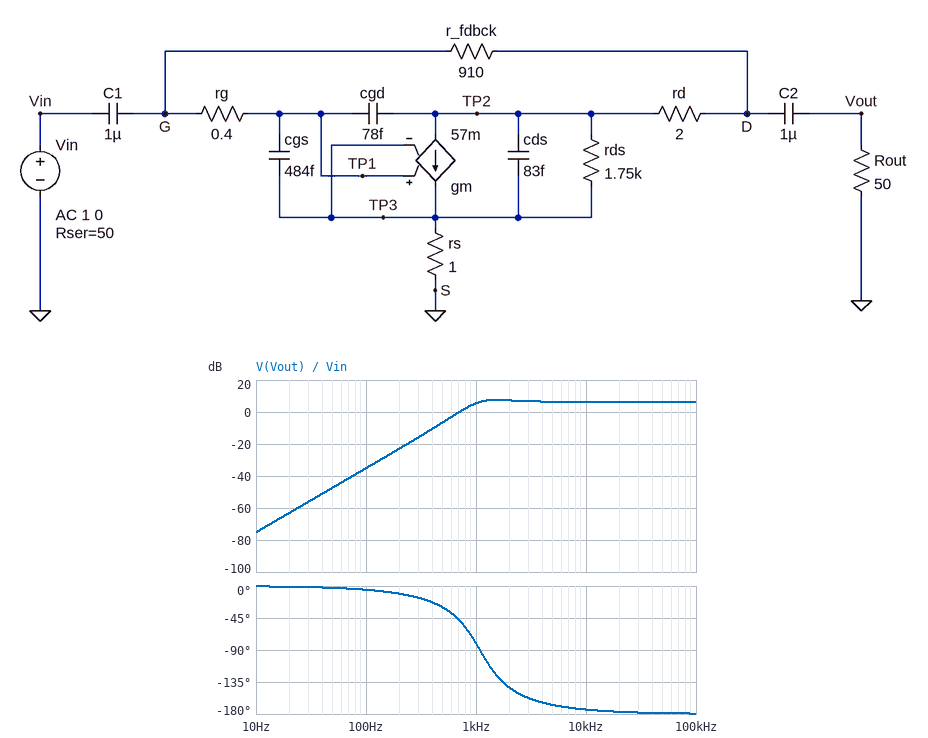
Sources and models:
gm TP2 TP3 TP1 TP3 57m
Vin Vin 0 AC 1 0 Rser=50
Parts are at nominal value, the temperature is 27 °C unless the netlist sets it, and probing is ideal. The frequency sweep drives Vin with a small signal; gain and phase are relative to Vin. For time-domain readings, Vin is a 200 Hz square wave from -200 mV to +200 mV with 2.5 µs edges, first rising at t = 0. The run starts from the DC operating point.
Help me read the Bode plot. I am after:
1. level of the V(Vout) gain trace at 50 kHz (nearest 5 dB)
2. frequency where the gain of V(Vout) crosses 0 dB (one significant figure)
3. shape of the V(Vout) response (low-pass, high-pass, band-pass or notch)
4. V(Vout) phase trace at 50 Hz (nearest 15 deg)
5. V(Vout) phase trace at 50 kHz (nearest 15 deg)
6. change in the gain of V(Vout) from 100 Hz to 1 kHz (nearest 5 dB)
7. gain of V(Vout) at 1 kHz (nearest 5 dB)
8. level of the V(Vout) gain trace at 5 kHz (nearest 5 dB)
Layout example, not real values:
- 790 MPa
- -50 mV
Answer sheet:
- 5 dB
- 700 Hz
- high-pass
- 0 deg
- -180 deg
- 40 dB
- 5 dB
- 5 dB
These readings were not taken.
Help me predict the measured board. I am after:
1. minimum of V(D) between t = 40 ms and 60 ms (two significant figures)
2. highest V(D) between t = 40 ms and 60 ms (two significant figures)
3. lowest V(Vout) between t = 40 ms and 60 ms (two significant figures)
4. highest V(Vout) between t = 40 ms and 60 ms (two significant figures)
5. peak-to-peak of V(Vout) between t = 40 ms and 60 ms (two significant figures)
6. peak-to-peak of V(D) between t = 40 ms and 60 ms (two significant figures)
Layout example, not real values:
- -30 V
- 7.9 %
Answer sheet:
- -1.4 V
- 1.4 V
- -810 mV
- 810 mV
- 1.6 V
- 2.8 V
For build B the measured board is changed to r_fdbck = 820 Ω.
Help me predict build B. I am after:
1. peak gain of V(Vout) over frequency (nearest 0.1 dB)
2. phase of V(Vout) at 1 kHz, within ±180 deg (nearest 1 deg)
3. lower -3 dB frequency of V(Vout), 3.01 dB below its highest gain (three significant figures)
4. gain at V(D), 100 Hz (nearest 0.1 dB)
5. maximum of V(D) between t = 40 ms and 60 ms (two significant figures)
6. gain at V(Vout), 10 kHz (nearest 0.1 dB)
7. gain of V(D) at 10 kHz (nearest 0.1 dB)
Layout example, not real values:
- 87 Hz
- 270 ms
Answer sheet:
- 7.1 dB
- -77 deg
- 972 Hz
- -6.0 dB
- 1.3 V
- 6.1 dB
- 6.5 dB
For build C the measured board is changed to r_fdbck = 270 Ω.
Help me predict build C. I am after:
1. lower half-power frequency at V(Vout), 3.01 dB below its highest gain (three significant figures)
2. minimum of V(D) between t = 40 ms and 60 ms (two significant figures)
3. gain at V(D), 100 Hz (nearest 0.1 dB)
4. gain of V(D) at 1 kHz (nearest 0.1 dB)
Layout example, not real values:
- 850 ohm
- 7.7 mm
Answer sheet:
- 1.66 kHz
- -570 mV
- -16.1 dB
- 3.6 dB
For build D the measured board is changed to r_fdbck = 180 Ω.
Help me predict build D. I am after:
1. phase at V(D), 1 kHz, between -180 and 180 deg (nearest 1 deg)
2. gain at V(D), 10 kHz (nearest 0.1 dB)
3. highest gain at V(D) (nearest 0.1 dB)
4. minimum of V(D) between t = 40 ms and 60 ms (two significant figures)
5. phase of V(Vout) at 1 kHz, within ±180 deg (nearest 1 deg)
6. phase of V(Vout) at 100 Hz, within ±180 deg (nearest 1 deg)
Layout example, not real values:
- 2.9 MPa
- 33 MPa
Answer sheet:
- -124 deg
- 0.6 dB
- 2.7 dB
- -420 mV
- -51 deg
- -5 deg
